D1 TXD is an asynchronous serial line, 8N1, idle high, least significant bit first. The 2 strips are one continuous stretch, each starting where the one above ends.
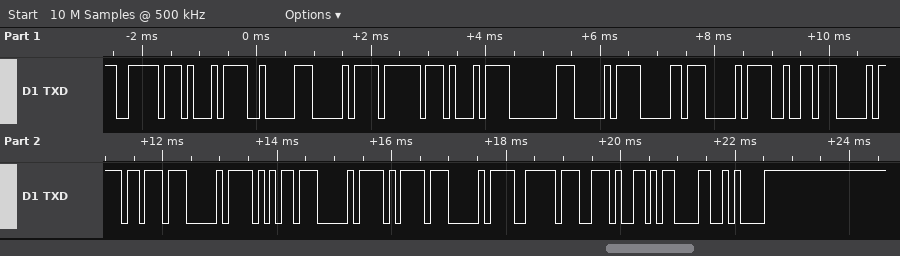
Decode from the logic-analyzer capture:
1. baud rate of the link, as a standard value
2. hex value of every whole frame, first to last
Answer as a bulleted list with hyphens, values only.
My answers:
- 9600 baud
- BE D1 82 D0 BF D1 80 D0 B0 D0 B2 D0 BB D0 B5 D0 BD D0 BE 2E 0D 0A
